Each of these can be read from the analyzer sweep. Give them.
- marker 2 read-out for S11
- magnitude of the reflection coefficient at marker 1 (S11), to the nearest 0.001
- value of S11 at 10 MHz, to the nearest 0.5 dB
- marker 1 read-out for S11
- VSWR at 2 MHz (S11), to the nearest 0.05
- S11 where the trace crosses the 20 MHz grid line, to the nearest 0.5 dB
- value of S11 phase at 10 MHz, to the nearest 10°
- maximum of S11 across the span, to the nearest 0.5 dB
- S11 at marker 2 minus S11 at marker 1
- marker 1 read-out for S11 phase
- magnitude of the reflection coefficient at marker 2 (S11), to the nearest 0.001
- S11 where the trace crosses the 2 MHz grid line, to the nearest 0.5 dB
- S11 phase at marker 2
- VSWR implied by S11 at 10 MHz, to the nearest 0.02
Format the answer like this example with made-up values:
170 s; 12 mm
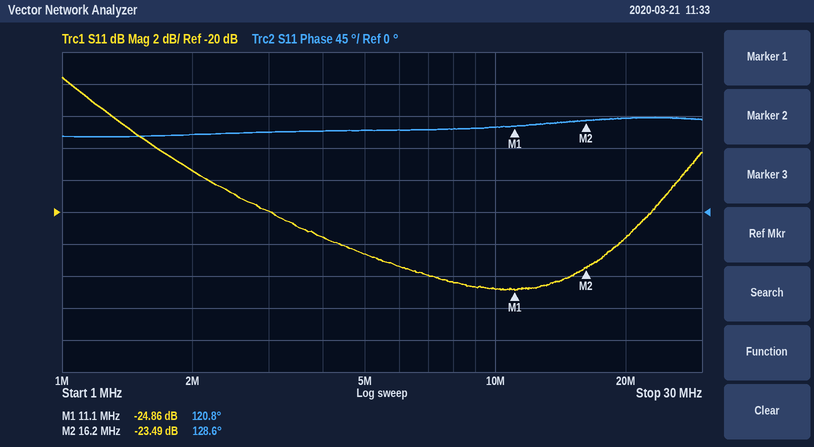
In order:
-23.49 dB; 0.057; -25.0 dB; -24.86 dB; 1.30; -21.5 dB; 120°; -11.5 dB; 1.37 dB; 120.8°; 0.067; -17.5 dB; 128.6°; 1.12
